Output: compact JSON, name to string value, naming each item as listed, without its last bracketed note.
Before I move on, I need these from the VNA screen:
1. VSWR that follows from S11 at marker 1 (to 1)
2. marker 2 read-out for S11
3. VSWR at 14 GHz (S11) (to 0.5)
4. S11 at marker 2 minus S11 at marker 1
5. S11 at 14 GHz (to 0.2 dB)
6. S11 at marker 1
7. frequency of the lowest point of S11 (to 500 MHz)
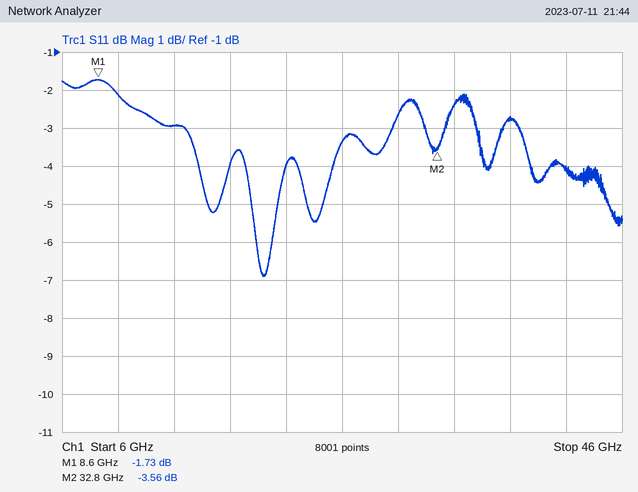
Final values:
{"VSWR that follows from S11 at marker 1": "10", "marker 2 read-out for S11": "-3.56 dB", "VSWR at 14 GHz (S11)": "6.0", "S11 at marker 2 minus S11 at marker 1": "-1.83 dB", "S11 at 14 GHz": "-3.0 dB", "S11 at marker 1": "-1.73 dB", "frequency of the lowest point of S11": "20.5 GHz"}
